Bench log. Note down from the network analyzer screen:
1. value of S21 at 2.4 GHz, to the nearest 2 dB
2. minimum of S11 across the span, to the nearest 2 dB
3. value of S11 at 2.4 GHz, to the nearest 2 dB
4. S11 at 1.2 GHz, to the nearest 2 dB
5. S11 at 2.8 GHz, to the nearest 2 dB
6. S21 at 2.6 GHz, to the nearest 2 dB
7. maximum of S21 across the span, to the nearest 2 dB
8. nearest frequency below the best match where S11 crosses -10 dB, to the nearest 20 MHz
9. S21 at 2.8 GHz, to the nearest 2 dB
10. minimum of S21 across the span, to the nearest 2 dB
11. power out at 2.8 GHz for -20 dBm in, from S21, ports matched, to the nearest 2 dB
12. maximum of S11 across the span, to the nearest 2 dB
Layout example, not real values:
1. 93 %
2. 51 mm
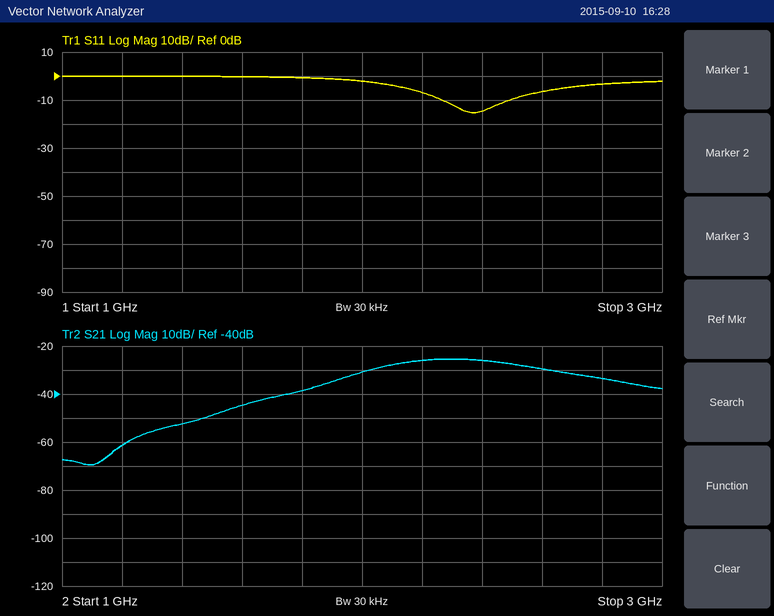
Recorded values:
1. -26 dB
2. -16 dB
3. -14 dB
4. 0 dB
5. -4 dB
6. -30 dB
7. -26 dB
8. 2.26 GHz
9. -34 dB
10. -70 dB
11. -54 dBm
12. 0 dB
